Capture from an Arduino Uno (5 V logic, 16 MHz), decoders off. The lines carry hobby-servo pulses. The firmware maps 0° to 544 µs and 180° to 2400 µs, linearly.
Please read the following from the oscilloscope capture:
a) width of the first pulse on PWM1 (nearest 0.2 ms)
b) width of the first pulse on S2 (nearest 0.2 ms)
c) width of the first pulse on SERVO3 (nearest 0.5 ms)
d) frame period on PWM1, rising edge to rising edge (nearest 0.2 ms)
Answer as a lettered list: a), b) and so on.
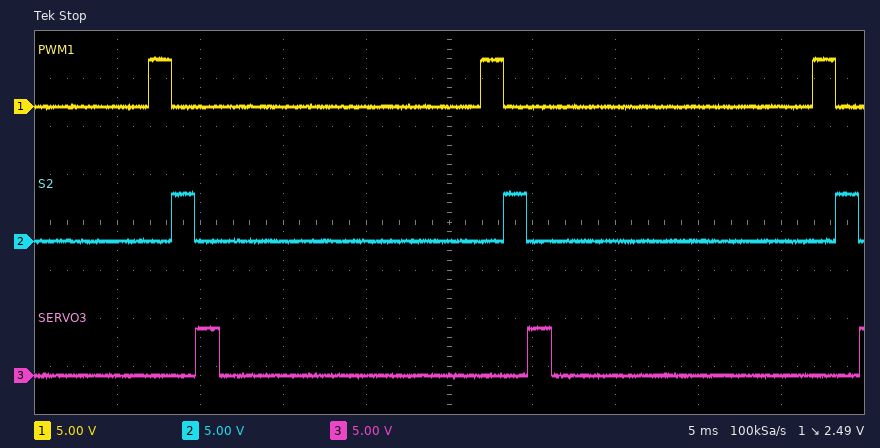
a) 1.4 ms
b) 1.4 ms
c) 1.5 ms
d) 20.0 ms
